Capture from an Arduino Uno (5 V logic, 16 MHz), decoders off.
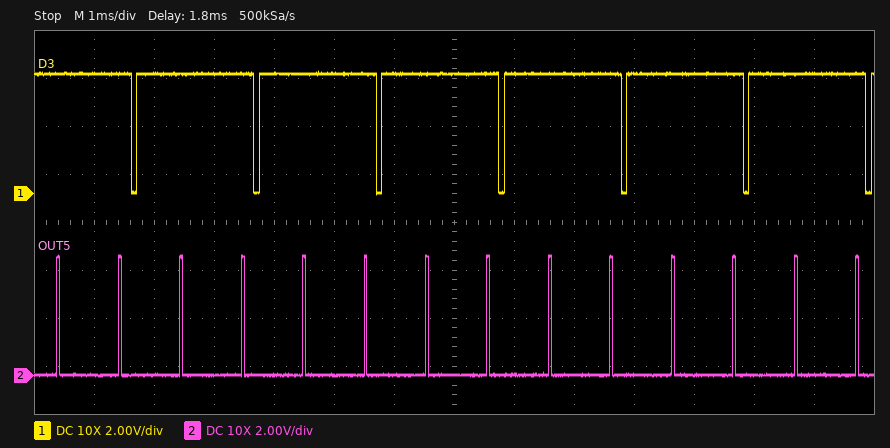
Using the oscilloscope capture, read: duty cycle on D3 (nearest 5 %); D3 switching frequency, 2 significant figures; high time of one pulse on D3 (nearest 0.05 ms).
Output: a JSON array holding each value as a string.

["95 %", "490 Hz", "1.95 ms"]
